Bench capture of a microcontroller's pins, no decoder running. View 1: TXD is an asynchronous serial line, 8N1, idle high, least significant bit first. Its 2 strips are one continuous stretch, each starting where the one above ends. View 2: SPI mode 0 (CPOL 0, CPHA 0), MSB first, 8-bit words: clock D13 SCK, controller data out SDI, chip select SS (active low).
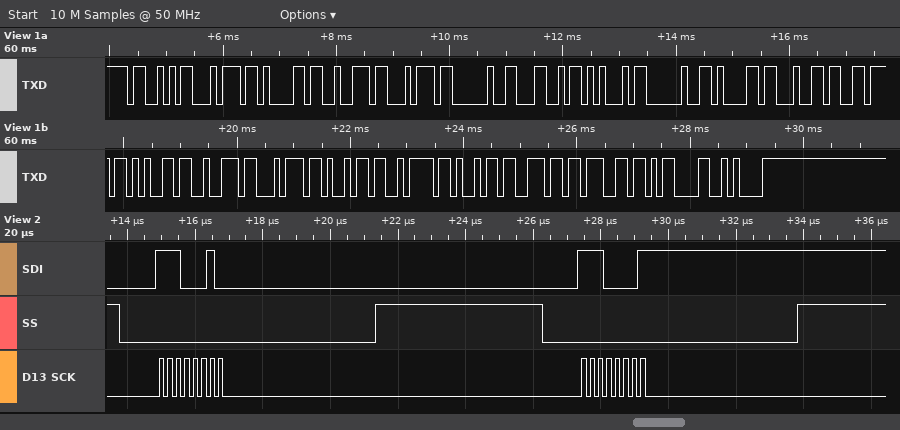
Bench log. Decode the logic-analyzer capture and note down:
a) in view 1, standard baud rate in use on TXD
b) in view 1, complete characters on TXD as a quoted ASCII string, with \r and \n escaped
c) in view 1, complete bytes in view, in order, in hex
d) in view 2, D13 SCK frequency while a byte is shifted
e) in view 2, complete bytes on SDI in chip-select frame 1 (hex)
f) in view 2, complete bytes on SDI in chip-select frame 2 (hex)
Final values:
9600 baud
"Start LE advertizing\r\n"
53 74 61 72 74 20 4C 45 20 61 64 76 65 72 74 69 7A 69 6E 67 0D 0A
4 MHz
0xE2
0xE1
